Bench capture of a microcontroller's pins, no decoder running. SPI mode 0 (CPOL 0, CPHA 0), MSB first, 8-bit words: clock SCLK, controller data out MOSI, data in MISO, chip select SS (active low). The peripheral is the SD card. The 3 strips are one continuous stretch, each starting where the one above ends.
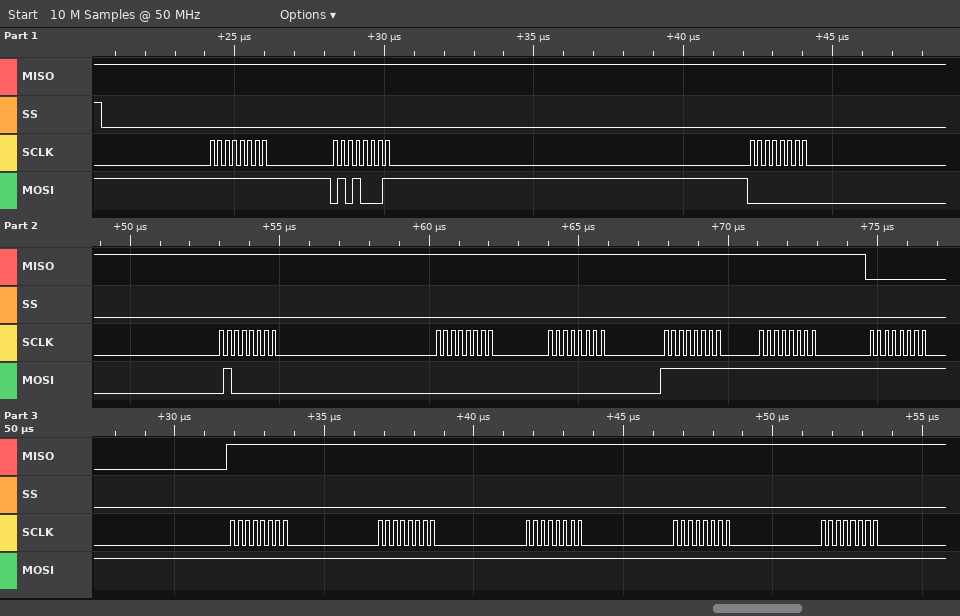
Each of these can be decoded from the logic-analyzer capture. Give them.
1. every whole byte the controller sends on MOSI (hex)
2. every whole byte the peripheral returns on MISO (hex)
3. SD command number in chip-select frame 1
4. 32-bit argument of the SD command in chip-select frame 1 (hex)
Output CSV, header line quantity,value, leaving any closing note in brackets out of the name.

quantity,value
every whole byte the controller sends on MOSI,0xFF 0x51 0x00 0x40 0x00 0x00 0xFF 0xFF 0xFF 0xFF 0xFF 0xFF 0xFF 0xFF
every whole byte the peripheral returns on MISO,0xFF 0xFF 0xFF 0xFF 0xFF 0xFF 0xFF 0xFF 0x00 0xFF 0xFF 0xFF 0xFF 0xFF
SD command number in chip-select frame 1,CMD17
32-bit argument of the SD command in chip-select frame 1,0x00400000
